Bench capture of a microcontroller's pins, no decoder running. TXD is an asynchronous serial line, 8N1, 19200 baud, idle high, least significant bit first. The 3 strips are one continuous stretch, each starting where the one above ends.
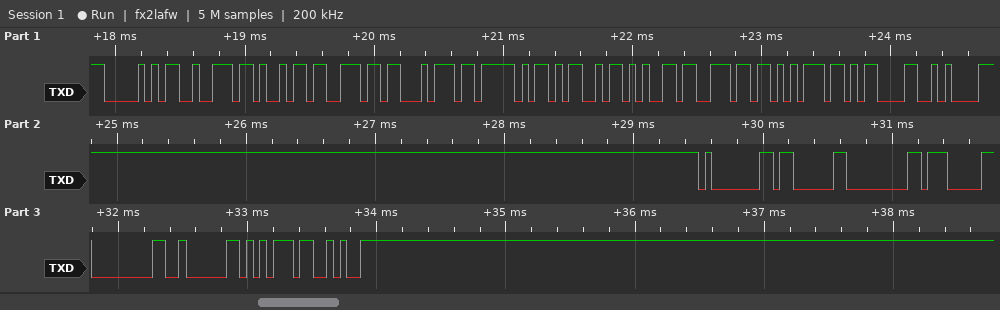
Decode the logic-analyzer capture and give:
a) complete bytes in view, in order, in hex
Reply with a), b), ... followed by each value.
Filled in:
a) 50 72 69 6E 74 5F 4D 65 6E 75 0D 0A 01 03 00 07 00 02 75 CA
